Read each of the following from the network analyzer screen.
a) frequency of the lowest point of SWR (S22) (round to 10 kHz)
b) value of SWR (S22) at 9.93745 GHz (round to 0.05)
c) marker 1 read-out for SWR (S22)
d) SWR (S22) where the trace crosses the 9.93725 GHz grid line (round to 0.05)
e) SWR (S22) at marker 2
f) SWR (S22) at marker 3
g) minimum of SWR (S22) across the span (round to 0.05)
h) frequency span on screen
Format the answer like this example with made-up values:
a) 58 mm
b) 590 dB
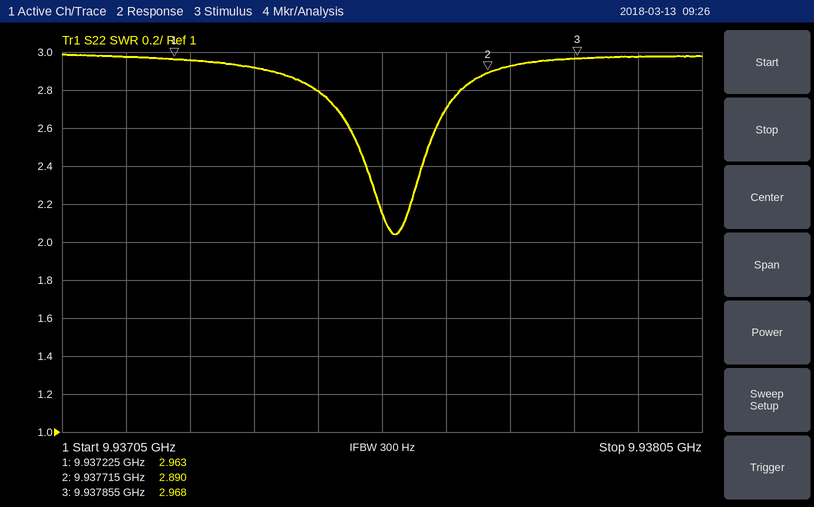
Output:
a) 9.93757 GHz
b) 2.80
c) 2.963
d) 2.95
e) 2.890
f) 2.968
g) 2.05
h) 1 MHz
